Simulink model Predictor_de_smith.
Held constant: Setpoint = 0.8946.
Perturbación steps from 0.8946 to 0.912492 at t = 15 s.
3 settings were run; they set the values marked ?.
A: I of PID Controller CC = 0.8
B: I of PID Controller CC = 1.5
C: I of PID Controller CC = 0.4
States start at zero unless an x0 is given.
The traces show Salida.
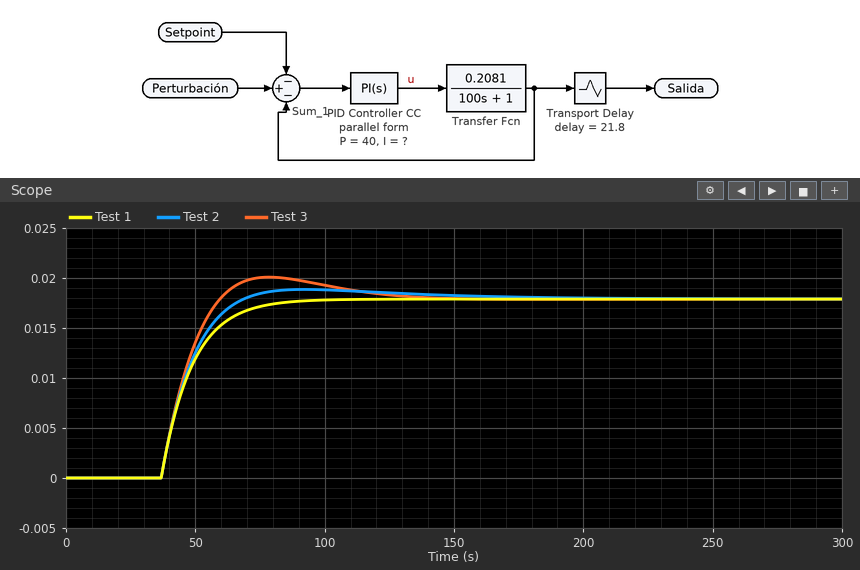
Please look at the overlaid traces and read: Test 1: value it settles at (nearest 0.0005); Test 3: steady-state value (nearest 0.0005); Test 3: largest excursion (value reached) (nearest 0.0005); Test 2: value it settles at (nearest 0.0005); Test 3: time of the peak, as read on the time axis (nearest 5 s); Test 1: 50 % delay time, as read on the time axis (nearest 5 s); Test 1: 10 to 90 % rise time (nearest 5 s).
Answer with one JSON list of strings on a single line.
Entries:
["0.0180", "0.0180", "0.0200", "0.0180", "80 s", "45 s", "25 s"]
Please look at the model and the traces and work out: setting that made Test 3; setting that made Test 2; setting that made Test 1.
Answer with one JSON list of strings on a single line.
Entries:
["B", "A", "C"]
